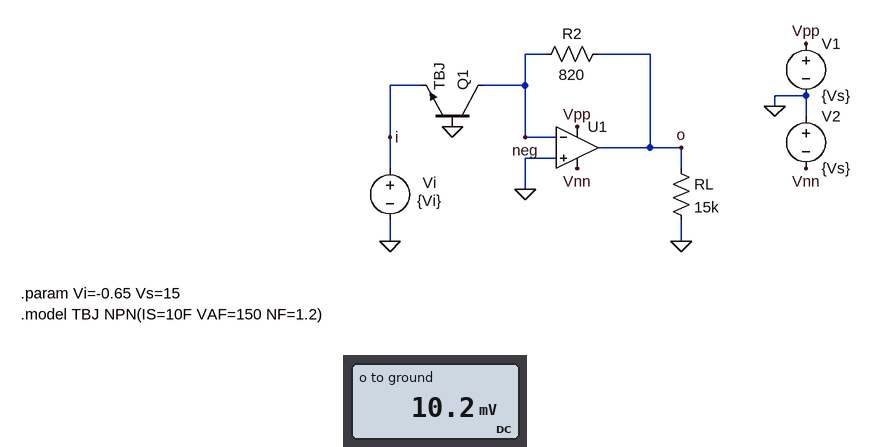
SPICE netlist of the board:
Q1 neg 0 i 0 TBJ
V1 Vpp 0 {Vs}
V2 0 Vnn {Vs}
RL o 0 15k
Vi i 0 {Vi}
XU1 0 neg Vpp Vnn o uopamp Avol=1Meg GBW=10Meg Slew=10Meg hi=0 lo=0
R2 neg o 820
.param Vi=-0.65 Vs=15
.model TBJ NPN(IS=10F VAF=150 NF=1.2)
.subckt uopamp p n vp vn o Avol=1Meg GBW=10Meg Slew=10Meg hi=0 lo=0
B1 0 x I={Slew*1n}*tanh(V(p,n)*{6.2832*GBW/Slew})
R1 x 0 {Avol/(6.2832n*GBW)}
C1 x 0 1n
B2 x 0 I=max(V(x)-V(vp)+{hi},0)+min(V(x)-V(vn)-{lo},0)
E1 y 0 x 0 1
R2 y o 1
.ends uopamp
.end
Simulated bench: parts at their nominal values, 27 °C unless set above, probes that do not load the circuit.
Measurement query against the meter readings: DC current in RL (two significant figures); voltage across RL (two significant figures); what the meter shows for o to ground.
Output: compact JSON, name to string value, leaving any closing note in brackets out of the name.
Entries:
{"DC current in RL": "680 nA", "voltage across RL": "10 mV", "what the meter shows for o to ground": "10.2 mV"}
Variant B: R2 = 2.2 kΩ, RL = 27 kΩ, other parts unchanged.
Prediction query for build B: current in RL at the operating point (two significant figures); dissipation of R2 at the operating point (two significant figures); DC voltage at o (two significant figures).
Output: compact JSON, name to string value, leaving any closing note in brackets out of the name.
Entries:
{"current in RL at the operating point": "1.0 µA", "dissipation of R2 at the operating point": "340 nW", "DC voltage at o": "27 mV"}
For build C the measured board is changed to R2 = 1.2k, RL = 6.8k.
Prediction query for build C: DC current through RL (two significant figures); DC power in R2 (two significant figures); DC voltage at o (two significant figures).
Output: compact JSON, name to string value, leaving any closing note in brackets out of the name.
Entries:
{"DC current through RL": "2.2 µA", "DC power in R2": "190 nW", "DC voltage at o": "15 mV"}
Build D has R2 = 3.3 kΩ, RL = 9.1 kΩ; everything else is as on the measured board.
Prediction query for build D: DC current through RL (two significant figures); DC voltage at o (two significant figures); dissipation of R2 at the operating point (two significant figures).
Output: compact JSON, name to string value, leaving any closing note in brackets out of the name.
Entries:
{"DC current through RL": "4.5 µA", "DC voltage at o": "41 mV", "dissipation of R2 at the operating point": "510 nW"}
